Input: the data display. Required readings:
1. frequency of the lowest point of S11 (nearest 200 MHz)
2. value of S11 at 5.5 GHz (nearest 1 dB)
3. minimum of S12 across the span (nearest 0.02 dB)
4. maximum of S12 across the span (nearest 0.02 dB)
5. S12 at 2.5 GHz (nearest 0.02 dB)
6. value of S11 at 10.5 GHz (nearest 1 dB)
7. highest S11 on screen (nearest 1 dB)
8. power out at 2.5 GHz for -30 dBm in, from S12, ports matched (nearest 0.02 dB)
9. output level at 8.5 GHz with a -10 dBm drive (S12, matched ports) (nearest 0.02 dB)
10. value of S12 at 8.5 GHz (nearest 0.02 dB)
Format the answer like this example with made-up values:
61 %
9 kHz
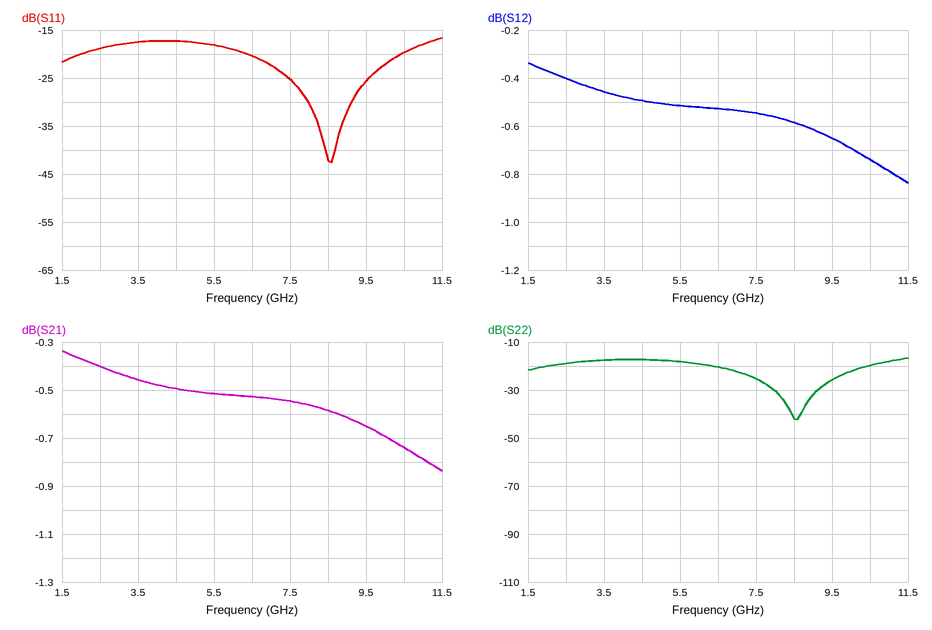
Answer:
8.6 GHz
-18 dB
-0.84 dB
-0.34 dB
-0.40 dB
-20 dB
-17 dB
-30.40 dBm
-10.58 dBm
-0.58 dB
